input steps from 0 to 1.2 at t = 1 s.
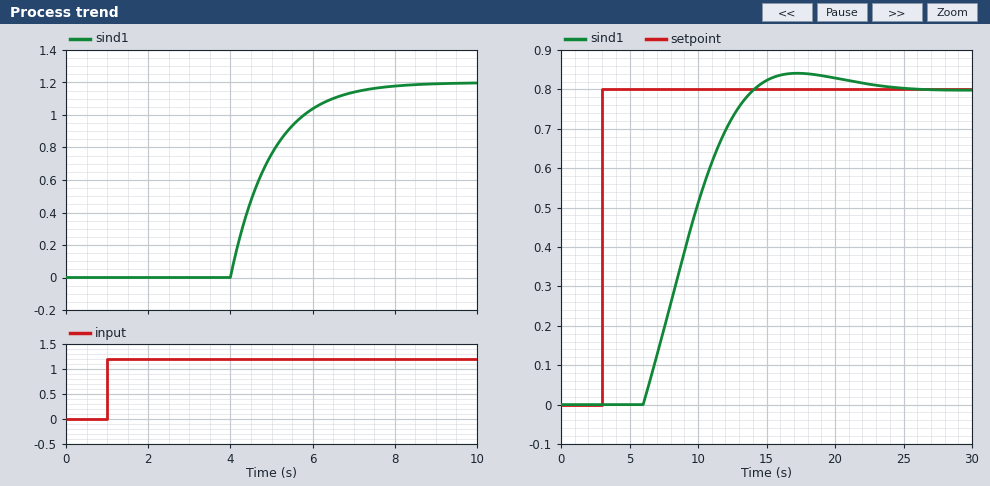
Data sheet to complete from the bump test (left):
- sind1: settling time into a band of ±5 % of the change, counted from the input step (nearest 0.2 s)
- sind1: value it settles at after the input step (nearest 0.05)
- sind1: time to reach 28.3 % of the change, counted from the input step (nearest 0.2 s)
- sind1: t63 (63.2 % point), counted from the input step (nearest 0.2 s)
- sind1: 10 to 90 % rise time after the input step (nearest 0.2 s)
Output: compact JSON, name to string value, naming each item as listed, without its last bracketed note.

{"sind1: settling time into a band of ±5 % of the change, counted from the input step": "6.0 s", "sind1: value it settles at after the input step": "1.20", "sind1: time to reach 28.3 % of the change, counted from the input step": "3.4 s", "sind1: t63 (63.2 % point), counted from the input step": "4.0 s", "sind1: 10 to 90 % rise time after the input step": "2.2 s"}
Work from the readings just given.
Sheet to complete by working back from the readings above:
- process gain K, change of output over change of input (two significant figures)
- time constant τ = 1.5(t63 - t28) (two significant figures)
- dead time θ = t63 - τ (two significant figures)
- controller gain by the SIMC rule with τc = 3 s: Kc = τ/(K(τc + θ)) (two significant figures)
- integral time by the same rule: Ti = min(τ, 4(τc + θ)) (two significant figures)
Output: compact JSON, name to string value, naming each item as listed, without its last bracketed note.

{"process gain K, change of output over change of input": "1.0", "time constant τ = 1.5(t63 - t28)": "0.90 s", "dead time θ = t63 - τ": "3.1 s", "controller gain by the SIMC rule with τc = 3 s: Kc = τ/(K(τc + θ))": "0.15", "integral time by the same rule: Ti = min(τ, 4(τc + θ))": "0.90 s"}
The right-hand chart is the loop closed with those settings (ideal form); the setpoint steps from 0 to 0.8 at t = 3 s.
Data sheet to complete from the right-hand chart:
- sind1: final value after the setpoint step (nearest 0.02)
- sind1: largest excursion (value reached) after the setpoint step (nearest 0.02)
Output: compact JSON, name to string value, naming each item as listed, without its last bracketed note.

{"sind1: final value after the setpoint step": "0.80", "sind1: largest excursion (value reached) after the setpoint step": "0.84"}
